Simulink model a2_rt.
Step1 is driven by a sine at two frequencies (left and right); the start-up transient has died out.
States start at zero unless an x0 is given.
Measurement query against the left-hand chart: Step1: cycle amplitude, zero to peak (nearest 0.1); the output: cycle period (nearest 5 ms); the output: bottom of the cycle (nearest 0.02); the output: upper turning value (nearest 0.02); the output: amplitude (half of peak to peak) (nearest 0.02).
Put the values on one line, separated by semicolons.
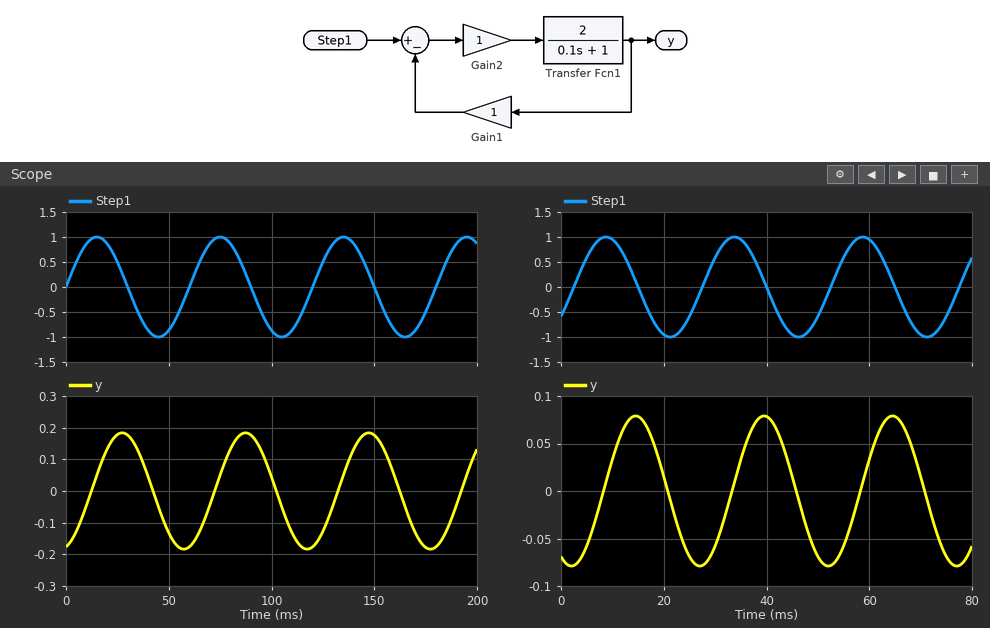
1.0; 60 ms; -0.18; 0.18; 0.18
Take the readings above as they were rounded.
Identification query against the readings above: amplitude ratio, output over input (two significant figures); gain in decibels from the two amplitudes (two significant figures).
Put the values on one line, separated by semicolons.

0.18; -15 dB
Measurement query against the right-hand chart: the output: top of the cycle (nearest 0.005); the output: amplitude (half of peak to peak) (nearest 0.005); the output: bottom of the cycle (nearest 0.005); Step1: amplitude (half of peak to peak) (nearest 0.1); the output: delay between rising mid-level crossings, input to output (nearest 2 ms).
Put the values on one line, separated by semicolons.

0.080; 0.080; -0.080; 1.0; 6 ms
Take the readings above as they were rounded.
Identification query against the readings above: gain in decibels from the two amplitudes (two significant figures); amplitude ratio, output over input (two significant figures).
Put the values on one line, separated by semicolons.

-22 dB; 0.080
